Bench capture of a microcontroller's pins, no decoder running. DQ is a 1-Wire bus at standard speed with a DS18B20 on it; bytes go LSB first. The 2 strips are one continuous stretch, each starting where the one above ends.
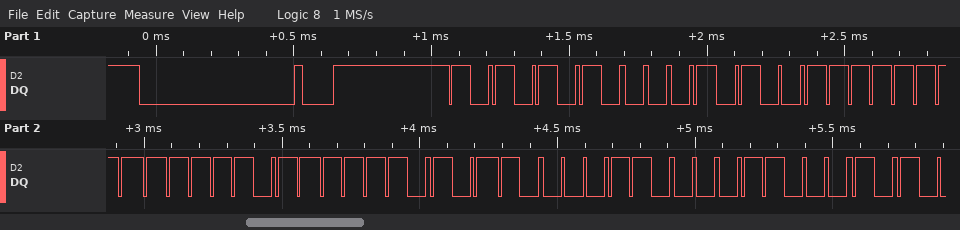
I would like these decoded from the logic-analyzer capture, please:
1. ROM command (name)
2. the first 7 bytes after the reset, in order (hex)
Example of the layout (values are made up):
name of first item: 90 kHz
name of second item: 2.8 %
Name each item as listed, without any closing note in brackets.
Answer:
ROM command: Match ROM
the first 7 bytes after the reset, in order: 55 28 FF DF AF 61 18
